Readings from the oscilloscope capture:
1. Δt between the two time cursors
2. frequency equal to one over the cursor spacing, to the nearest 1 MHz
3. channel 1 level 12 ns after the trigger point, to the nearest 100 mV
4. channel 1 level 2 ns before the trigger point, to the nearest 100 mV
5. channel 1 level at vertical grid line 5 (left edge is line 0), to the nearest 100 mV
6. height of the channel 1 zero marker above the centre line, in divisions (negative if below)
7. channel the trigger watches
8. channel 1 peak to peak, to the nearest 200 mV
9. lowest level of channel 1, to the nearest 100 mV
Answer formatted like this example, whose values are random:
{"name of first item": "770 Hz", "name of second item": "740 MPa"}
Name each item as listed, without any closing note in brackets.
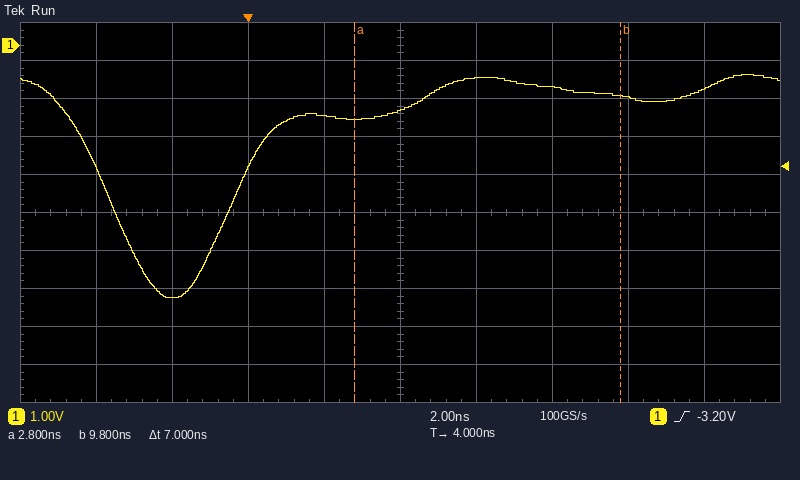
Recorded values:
{"Δt between the two time cursors": "7 ns", "frequency equal to one over the cursor spacing, to the nearest 1 MHz": "143 MHz", "channel 1 level 12 ns after the trigger point, to the nearest 100 mV": "-1.2 V", "channel 1 level 2 ns before the trigger point, to the nearest 100 mV": "-6.6 V", "channel 1 level at vertical grid line 5 (left edge is line 0), to the nearest 100 mV": "-1.7 V", "height of the channel 1 zero marker above the centre line, in divisions": "+4.4 div", "channel the trigger watches": "channel 1", "channel 1 peak to peak, to the nearest 200 mV": "5.8 V", "lowest level of channel 1, to the nearest 100 mV": "-6.6 V"}
